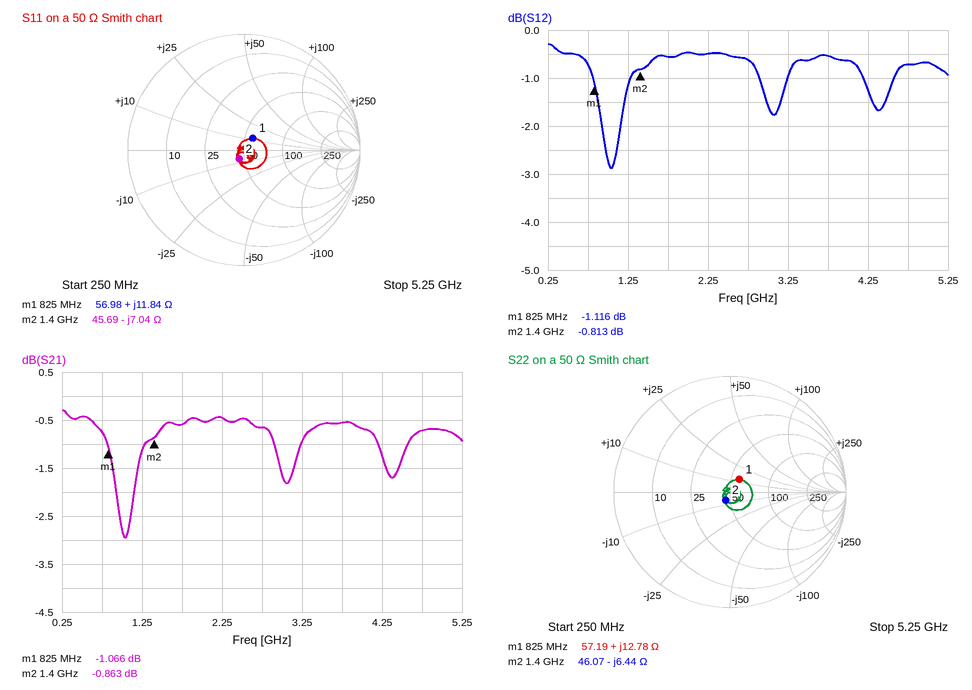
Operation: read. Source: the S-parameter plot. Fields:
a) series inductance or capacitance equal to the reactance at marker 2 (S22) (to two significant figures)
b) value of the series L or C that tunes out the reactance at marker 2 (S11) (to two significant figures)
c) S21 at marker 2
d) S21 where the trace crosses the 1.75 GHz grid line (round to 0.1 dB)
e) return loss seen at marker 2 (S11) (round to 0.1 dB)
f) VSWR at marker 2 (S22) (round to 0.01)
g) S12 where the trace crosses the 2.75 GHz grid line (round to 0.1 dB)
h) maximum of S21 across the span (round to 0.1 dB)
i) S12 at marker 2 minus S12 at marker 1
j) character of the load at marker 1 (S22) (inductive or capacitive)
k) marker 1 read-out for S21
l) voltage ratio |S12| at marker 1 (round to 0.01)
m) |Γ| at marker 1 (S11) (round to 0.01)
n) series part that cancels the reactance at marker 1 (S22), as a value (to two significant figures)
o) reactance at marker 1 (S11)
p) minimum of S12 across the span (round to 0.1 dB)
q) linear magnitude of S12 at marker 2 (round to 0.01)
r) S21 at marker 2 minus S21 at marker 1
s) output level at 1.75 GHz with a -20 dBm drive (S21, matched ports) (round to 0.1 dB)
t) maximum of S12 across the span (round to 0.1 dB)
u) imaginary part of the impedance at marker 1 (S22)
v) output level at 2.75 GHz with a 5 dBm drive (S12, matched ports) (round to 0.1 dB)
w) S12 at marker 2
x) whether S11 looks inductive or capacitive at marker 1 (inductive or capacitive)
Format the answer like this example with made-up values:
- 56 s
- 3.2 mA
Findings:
- 18 pF
- 800 pH
- -0.863 dB
- -0.6 dB
- 21.3 dB
- 1.17
- -0.6 dB
- -0.3 dB
- 0.303 dB
- inductive
- -1.066 dB
- 0.88
- 0.13
- 15 pF
- +11.84 Ω
- -2.9 dB
- 0.91
- 0.203 dB
- -20.6 dBm
- -0.3 dB
- +12.78 Ω
- 4.4 dBm
- -0.813 dB
- inductive
